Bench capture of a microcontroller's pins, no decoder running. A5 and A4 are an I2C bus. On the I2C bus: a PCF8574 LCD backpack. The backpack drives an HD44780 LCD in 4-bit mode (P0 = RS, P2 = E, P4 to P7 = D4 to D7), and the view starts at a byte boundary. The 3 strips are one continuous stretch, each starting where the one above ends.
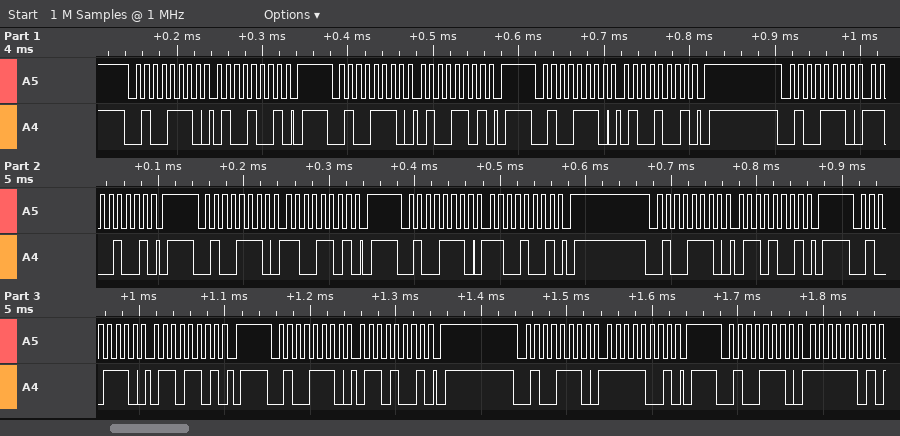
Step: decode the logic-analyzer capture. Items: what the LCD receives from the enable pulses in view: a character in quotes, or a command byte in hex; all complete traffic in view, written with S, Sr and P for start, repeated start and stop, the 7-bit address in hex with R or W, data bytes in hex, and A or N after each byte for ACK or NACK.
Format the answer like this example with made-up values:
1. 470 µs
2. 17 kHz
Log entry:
1. 'L'
2. S 27W A 49 A P S 27W A 4D A P S 27W A 49 A P S 27W A C9 A P S 27W A CD A P S 27W A C9 A P S 27W A 69 A P S 27W A 6D A P S 27W A 69 A P S 27W A F9 A P S 27W A FD A
